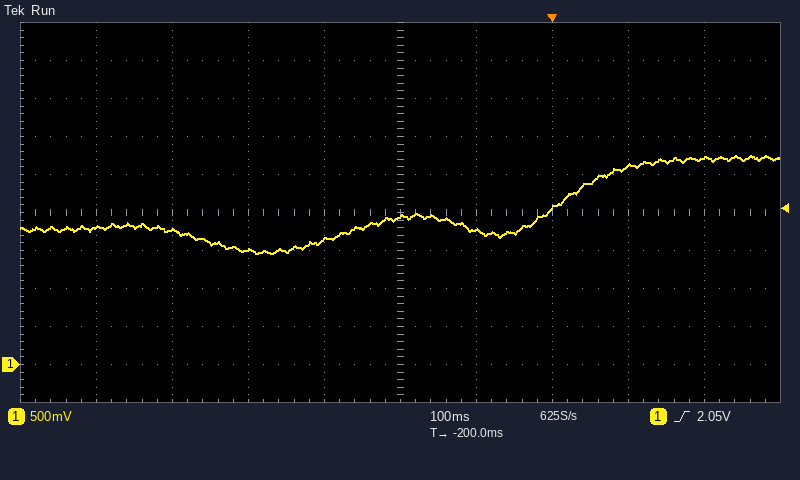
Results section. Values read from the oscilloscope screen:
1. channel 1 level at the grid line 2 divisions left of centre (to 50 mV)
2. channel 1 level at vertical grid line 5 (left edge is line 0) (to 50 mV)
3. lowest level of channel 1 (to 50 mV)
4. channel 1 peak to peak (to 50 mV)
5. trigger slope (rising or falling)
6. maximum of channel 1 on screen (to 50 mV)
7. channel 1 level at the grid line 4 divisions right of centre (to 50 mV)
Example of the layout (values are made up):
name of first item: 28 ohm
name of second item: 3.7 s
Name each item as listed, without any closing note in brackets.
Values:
channel 1 level at the grid line 2 divisions left of centre: 1.50 V
channel 1 level at vertical grid line 5 (left edge is line 0): 1.95 V
lowest level of channel 1: 1.45 V
channel 1 peak to peak: 1.30 V
trigger slope: rising
maximum of channel 1 on screen: 2.75 V
channel 1 level at the grid line 4 divisions right of centre: 2.70 V
